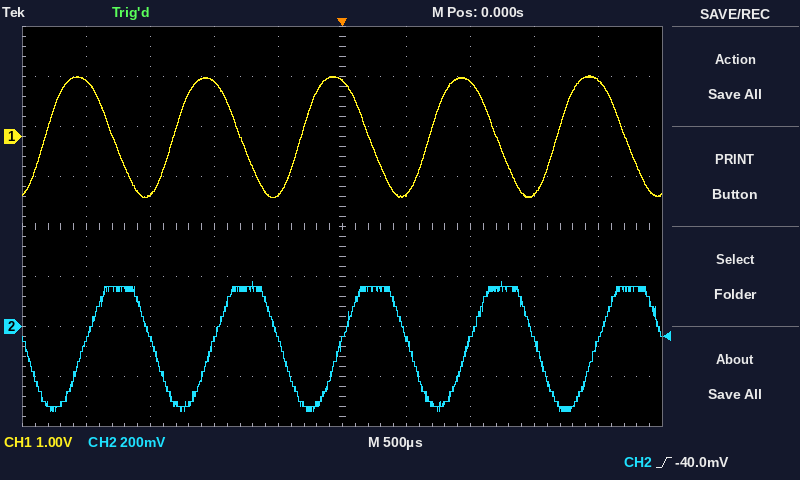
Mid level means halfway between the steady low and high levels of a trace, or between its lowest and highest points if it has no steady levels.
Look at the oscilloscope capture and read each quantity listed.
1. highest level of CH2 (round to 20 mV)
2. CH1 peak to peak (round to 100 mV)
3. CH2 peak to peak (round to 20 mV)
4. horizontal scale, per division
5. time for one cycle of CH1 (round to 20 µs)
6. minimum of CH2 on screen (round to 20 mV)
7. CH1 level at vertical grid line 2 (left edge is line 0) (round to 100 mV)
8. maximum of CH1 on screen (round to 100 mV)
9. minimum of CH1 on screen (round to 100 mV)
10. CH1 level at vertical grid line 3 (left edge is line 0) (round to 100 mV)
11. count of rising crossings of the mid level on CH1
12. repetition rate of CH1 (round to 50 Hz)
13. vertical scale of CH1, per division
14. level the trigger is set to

180 mV
2.4 V
520 mV
500 µs
1.00 ms
-340 mV
-1.2 V
1.2 V
-1.2 V
1.1 V
5
1.00 kHz
1 V
-40.0 mV
